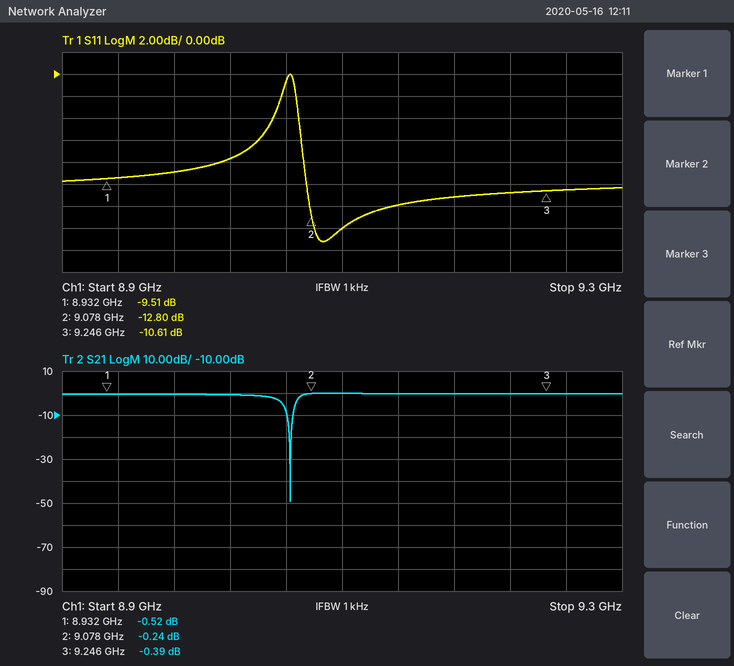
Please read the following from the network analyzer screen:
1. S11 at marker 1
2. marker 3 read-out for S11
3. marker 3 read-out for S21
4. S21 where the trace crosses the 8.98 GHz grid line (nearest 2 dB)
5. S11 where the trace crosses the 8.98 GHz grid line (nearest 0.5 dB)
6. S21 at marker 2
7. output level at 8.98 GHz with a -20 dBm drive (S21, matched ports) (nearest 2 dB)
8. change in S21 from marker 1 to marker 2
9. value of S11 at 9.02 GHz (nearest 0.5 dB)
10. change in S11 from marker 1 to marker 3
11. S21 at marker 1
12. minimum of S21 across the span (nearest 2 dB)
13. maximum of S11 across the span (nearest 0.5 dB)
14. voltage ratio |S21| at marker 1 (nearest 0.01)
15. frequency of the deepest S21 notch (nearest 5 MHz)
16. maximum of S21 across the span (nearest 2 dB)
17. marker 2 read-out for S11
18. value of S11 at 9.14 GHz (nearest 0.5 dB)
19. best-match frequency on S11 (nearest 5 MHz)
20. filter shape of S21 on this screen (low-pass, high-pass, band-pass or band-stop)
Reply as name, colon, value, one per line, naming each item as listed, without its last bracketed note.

S11 at marker 1: -9.51 dB
marker 3 read-out for S11: -10.61 dB
marker 3 read-out for S21: -0.39 dB
S21 where the trace crosses the 8.98 GHz grid line: 0 dB
S11 where the trace crosses the 8.98 GHz grid line: -9.0 dB
S21 at marker 2: -0.24 dB
output level at 8.98 GHz with a -20 dBm drive (S21, matched ports): -20 dBm
change in S21 from marker 1 to marker 2: 0.28 dB
value of S11 at 9.02 GHz: -7.5 dB
change in S11 from marker 1 to marker 3: -1.10 dB
S21 at marker 1: -0.52 dB
minimum of S21 across the span: -50 dB
maximum of S11 across the span: 0.0 dB
voltage ratio |S21| at marker 1: 0.94
frequency of the deepest S21 notch: 9.065 GHz
maximum of S21 across the span: 0 dB
marker 2 read-out for S11: -12.80 dB
value of S11 at 9.14 GHz: -12.0 dB
best-match frequency on S11: 9.085 GHz
filter shape of S21 on this screen: band-stop
